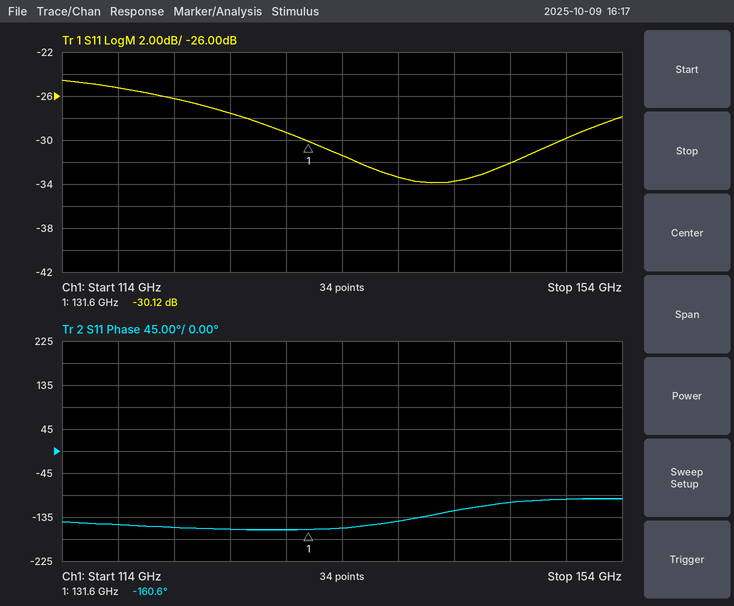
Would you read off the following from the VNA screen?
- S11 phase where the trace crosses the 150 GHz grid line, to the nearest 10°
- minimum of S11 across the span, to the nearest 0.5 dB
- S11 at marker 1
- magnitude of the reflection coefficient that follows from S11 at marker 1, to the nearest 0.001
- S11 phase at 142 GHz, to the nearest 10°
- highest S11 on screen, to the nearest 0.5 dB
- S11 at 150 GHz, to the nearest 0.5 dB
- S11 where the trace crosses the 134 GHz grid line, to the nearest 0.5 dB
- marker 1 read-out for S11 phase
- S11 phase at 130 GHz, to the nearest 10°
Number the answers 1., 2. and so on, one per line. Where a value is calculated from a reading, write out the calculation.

1. -100°
2. -34.0 dB
3. -30.12 dB
4. 10^(-30.12/20) ≈ 0.031
5. -120°
6. -24.5 dB
7. -30.0 dB
8. -31.5 dB
9. -160.6°
10. -160°
